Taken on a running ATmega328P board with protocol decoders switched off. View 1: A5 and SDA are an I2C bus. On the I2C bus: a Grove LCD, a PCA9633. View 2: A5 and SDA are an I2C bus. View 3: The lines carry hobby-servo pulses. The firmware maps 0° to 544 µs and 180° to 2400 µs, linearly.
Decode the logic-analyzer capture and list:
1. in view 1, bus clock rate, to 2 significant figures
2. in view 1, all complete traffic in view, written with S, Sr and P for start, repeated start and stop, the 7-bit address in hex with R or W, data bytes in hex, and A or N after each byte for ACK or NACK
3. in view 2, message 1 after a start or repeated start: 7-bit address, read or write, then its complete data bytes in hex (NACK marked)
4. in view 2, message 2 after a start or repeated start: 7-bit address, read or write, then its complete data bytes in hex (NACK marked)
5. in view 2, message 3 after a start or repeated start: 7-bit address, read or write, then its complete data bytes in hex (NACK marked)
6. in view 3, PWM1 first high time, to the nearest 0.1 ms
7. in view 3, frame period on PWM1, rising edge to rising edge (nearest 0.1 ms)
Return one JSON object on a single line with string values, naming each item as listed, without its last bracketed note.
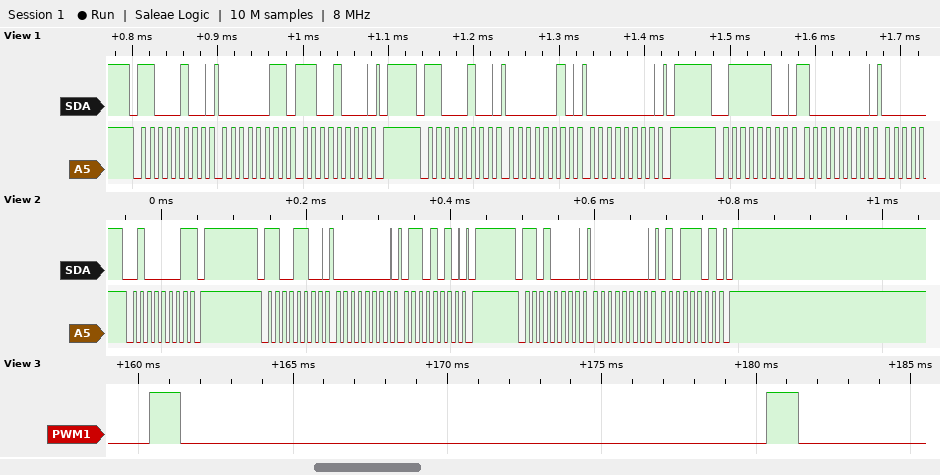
{"in view 1, bus clock rate, to 2 significant figures": "100 kHz", "in view 1, all complete traffic in view, written with S, Sr and P for start, repeated start and stop, the 7-bit address in hex with R or W, data bytes in hex, and A or N after each byte for ACK or NACK": "S 62W A 03 A C8 A P S 62W A 02 A 00 A P S 3EW A 80 A", "in view 2, message 1 after a start or repeated start: 7-bit address, read or write, then its complete data bytes in hex": "0x20 read NACK", "in view 2, message 2 after a start or repeated start: 7-bit address, read or write, then its complete data bytes in hex": "0x66 write: 00 6A", "in view 2, message 3 after a start or repeated start: 7-bit address, read or write, then its complete data bytes in hex": "0x68 write: 00 5D", "in view 3, PWM1 first high time, to the nearest 0.1 ms": "1.0 ms", "in view 3, frame period on PWM1, rising edge to rising edge": "20.0 ms"}
